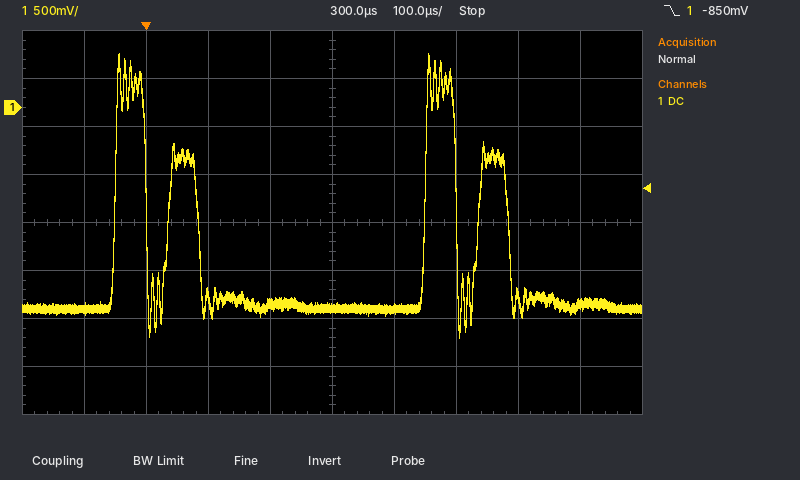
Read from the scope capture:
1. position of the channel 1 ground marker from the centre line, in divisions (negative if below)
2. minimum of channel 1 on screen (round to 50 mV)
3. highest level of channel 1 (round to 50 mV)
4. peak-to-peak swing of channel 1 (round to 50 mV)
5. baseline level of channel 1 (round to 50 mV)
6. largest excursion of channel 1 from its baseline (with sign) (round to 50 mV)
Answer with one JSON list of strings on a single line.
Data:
["+2.4 div", "-2.40 V", "550 mV", "2.95 V", "-2.10 V", "+2.65 V"]
